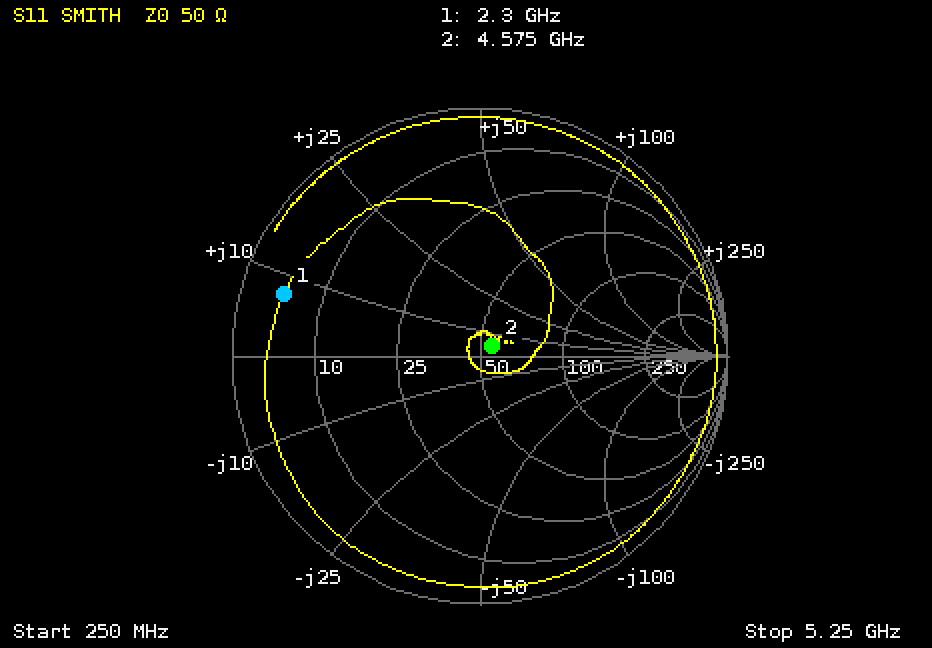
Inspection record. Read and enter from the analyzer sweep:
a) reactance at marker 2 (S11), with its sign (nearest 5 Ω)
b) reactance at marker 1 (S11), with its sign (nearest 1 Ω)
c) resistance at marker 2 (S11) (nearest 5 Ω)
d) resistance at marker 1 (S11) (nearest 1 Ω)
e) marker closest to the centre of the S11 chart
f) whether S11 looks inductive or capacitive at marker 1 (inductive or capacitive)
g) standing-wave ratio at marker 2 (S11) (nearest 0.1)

+5 Ω
+8 Ω
55 Ω
5 Ω
marker 2
inductive
1.1
